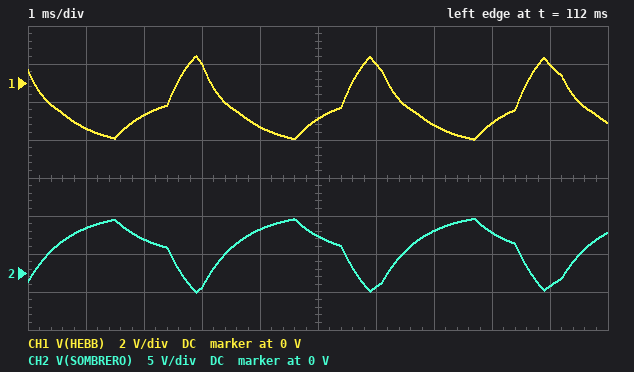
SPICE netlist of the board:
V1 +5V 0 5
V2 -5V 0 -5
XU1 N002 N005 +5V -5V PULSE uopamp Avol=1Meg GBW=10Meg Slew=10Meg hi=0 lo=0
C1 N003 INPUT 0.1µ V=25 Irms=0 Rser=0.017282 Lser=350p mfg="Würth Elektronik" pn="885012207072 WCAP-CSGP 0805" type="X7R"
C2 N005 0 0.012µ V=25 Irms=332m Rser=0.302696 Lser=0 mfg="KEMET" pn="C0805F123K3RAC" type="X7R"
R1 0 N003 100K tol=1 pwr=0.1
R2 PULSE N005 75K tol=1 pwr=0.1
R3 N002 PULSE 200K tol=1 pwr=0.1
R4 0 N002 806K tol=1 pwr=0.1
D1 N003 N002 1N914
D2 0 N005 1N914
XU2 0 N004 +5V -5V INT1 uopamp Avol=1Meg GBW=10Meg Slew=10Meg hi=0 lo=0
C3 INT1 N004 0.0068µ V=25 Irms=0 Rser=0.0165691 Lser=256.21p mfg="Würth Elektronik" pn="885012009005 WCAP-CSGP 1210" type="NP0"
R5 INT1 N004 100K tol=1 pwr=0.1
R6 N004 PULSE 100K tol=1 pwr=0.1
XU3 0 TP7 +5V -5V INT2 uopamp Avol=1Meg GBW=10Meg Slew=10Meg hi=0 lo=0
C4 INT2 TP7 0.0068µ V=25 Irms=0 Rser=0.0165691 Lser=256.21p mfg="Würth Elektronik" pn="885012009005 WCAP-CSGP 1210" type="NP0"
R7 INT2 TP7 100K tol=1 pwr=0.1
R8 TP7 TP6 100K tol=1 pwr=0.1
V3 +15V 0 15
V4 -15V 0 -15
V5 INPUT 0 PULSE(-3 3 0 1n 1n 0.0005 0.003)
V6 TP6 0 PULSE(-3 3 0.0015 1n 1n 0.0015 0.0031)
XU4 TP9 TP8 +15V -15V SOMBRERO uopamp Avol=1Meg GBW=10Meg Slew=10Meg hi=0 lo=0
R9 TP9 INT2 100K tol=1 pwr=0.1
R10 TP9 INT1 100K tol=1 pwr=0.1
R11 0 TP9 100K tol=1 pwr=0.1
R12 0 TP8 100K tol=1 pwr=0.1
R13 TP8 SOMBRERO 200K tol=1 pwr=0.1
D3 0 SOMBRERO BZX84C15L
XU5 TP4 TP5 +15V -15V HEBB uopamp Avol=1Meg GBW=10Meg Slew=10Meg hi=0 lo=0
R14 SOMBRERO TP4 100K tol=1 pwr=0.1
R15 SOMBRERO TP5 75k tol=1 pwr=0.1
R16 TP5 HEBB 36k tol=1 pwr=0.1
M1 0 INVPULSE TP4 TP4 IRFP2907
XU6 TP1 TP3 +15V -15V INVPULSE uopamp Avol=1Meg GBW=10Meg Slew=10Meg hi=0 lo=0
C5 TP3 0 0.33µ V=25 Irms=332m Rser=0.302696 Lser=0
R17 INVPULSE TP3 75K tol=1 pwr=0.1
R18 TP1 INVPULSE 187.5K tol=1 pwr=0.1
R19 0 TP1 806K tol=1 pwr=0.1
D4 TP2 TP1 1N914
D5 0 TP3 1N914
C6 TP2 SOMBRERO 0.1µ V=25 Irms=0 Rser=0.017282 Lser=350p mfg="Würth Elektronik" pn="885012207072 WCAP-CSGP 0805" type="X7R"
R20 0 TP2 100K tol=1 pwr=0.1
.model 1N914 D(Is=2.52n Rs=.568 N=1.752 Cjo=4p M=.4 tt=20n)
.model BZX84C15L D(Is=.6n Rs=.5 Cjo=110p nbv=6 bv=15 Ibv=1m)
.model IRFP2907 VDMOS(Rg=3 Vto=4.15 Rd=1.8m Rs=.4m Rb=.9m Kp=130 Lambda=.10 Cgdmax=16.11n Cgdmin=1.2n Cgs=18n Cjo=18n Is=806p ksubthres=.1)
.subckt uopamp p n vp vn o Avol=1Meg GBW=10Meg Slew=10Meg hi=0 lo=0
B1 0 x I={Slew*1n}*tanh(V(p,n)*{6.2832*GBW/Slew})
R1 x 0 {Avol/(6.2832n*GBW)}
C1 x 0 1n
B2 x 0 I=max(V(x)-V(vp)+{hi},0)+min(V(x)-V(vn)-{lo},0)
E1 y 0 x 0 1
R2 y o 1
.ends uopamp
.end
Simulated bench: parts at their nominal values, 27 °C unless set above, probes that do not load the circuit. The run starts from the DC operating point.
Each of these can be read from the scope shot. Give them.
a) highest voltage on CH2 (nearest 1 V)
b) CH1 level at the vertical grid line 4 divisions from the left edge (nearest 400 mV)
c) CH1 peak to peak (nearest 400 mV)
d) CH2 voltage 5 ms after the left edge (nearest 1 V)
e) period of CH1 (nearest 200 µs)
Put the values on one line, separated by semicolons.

7 V; -2.4 V; 4.4 V; 5 V; 3.0 ms
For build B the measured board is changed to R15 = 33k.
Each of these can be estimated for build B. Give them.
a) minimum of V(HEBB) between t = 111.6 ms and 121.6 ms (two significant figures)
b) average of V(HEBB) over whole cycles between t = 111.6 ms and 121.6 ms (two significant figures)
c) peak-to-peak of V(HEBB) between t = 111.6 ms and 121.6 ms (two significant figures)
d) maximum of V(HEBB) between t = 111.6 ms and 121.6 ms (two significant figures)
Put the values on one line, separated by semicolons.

-7.2 V; -3.3 V; 10 V; 3.0 V
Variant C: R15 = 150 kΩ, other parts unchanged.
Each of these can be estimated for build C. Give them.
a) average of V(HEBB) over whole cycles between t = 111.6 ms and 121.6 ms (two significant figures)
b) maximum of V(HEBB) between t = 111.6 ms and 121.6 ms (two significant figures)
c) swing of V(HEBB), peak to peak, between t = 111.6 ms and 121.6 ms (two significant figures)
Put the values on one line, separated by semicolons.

-550 mV; 760 mV; 2.1 V
